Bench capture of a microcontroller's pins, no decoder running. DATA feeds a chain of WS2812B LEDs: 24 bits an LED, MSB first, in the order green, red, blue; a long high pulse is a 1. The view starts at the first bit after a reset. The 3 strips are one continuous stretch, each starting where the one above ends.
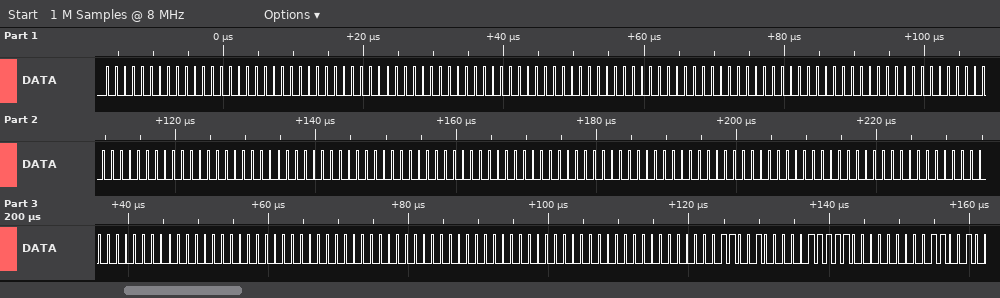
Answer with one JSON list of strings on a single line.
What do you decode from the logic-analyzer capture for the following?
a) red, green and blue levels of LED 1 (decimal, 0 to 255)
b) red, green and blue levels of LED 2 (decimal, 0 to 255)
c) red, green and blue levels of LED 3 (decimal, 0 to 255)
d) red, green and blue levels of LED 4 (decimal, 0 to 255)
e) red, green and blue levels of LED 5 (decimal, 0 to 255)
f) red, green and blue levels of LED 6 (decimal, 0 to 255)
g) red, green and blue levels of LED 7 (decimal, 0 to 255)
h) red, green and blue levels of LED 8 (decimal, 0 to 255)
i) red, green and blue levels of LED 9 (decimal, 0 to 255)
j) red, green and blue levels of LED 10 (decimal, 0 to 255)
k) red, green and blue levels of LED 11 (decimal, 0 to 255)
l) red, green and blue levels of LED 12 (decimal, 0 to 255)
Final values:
["0, 0, 0", "0, 0, 0", "0, 0, 0", "0, 0, 0", "0, 0, 0", "0, 0, 0", "0, 0, 0", "0, 0, 0", "0, 0, 0", "0, 0, 0", "0, 0, 0", "100, 0, 31"]
